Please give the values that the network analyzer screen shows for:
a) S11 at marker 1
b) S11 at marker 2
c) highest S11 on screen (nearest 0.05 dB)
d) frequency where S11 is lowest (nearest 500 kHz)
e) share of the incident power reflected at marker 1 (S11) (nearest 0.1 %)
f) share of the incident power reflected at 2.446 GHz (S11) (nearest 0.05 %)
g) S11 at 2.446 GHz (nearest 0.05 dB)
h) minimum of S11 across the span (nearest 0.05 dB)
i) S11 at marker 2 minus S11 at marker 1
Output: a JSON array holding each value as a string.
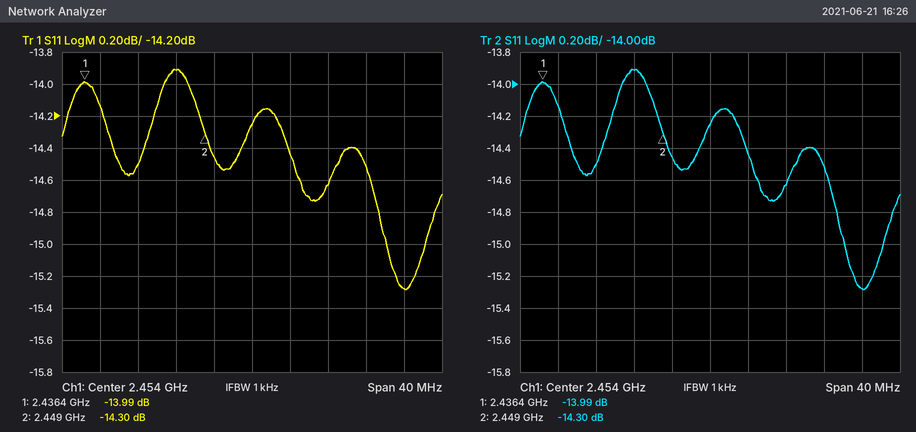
["-13.99 dB", "-14.30 dB", "-13.90 dB", "2.4700 GHz", "4.0 %", "4.05 %", "-13.90 dB", "-15.30 dB", "-0.31 dB"]
